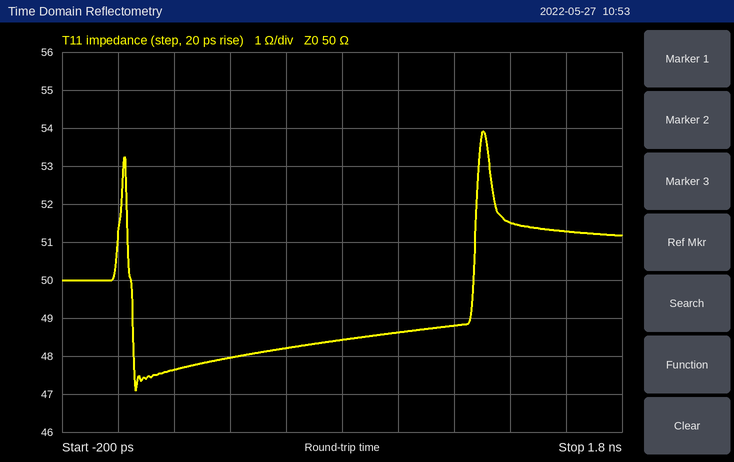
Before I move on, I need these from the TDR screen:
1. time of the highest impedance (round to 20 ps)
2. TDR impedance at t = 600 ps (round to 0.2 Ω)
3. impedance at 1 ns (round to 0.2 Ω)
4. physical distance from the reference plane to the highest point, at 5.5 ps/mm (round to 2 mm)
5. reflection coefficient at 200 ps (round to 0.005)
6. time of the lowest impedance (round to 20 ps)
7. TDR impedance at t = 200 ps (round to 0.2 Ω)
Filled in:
1.30 ns
48.2 Ω
48.6 Ω
118 mm
-0.025
60 ps
47.6 Ω
